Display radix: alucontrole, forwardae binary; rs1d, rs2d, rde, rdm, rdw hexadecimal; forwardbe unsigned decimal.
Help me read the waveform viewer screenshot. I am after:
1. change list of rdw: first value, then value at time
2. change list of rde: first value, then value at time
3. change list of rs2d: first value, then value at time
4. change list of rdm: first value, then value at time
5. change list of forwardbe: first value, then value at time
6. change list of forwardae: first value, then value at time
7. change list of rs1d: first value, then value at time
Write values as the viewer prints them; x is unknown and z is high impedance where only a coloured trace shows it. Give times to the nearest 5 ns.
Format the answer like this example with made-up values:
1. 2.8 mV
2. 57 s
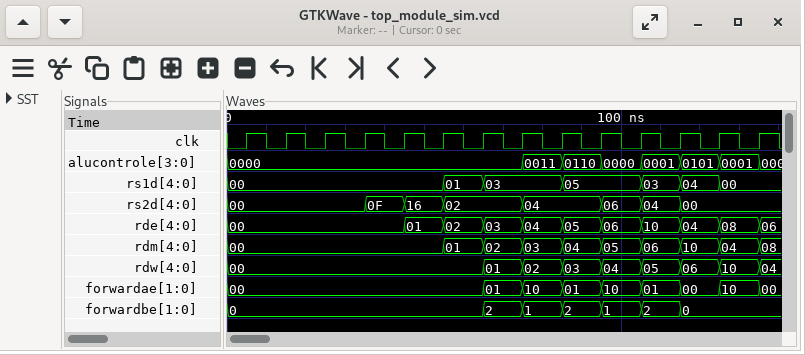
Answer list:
1. 00, 01 at 65 ns, 02 at 75 ns, 03 at 85 ns, 04 at 95 ns, 05 at 105 ns, 06 at 115 ns, 10 at 125 ns, 04 at 135 ns
2. 00, 01 at 45 ns, 02 at 55 ns, 03 at 65 ns, 04 at 75 ns, 05 at 85 ns, 06 at 95 ns, 10 at 105 ns, 04 at 115 ns, 08 at 125 ns, 06 at 135 ns
3. 00, 0F at 35 ns, 16 at 45 ns, 02 at 55 ns, 04 at 75 ns, 06 at 95 ns, 04 at 105 ns, 00 at 115 ns
4. 00, 01 at 55 ns, 02 at 65 ns, 03 at 75 ns, 04 at 85 ns, 05 at 95 ns, 06 at 105 ns, 10 at 115 ns, 04 at 125 ns, 08 at 135 ns
5. 0, 2 at 65 ns, 1 at 75 ns, 2 at 85 ns, 1 at 95 ns, 2 at 105 ns, 0 at 115 ns
6. 00, 01 at 65 ns, 10 at 75 ns, 01 at 85 ns, 10 at 95 ns, 01 at 105 ns, 00 at 115 ns, 10 at 125 ns, 00 at 135 ns
7. 00, 01 at 55 ns, 03 at 65 ns, 05 at 85 ns, 03 at 105 ns, 04 at 115 ns, 00 at 125 ns
